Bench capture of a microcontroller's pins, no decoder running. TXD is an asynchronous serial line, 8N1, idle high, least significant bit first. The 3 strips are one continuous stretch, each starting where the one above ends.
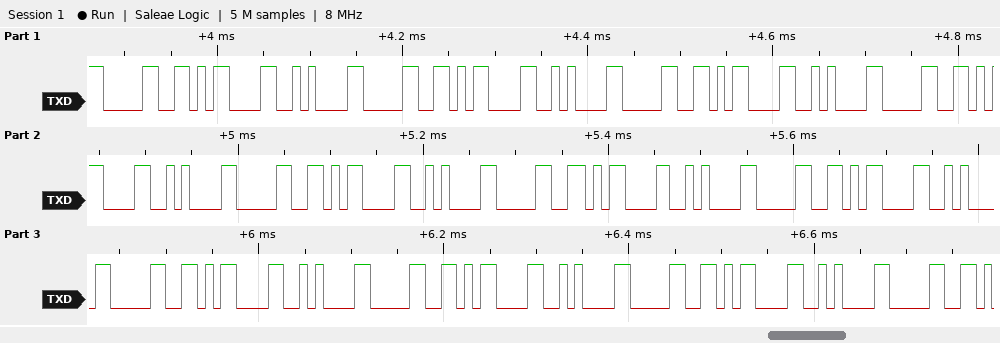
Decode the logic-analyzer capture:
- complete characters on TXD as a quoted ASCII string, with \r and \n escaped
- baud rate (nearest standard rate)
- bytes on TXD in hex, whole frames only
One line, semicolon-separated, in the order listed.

"0\r\n0\r\n0\r\n0\r\n0\r\n0\r\n0\r\n0\r\n0\r\n0\r\n0"; 115200 baud; 30 0D 0A 30 0D 0A 30 0D 0A 30 0D 0A 30 0D 0A 30 0D 0A 30 0D 0A 30 0D 0A 30 0D 0A 30 0D 0A 30
